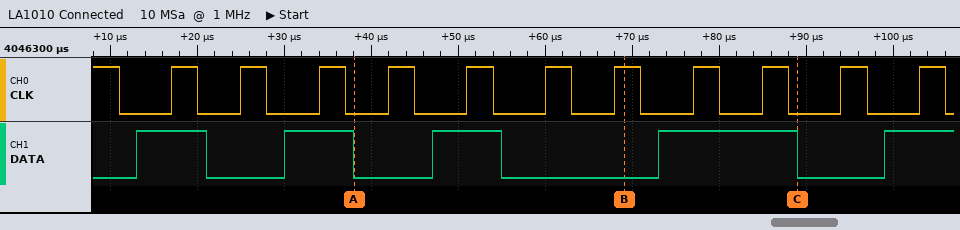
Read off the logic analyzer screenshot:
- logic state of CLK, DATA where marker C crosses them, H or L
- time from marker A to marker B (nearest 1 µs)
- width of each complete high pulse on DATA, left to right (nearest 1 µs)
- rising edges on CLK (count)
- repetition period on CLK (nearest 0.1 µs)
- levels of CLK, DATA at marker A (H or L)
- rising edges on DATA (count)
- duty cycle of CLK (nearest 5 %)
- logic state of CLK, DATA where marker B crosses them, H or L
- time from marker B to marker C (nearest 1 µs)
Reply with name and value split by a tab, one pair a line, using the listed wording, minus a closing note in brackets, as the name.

logic state of CLK, DATA where marker C crosses them, H or L	CLK=L, DATA=L
time from marker A to marker B	31 µs
width of each complete high pulse on DATA, left to right	8 µs, 8 µs, 8 µs, 16 µs
rising edges on CLK	11
repetition period on CLK	8.6 µs
levels of CLK, DATA at marker A	CLK=L, DATA=L
rising edges on DATA	5
duty cycle of CLK	35 %
logic state of CLK, DATA where marker B crosses them, H or L	CLK=H, DATA=L
time from marker B to marker C	20 µs
